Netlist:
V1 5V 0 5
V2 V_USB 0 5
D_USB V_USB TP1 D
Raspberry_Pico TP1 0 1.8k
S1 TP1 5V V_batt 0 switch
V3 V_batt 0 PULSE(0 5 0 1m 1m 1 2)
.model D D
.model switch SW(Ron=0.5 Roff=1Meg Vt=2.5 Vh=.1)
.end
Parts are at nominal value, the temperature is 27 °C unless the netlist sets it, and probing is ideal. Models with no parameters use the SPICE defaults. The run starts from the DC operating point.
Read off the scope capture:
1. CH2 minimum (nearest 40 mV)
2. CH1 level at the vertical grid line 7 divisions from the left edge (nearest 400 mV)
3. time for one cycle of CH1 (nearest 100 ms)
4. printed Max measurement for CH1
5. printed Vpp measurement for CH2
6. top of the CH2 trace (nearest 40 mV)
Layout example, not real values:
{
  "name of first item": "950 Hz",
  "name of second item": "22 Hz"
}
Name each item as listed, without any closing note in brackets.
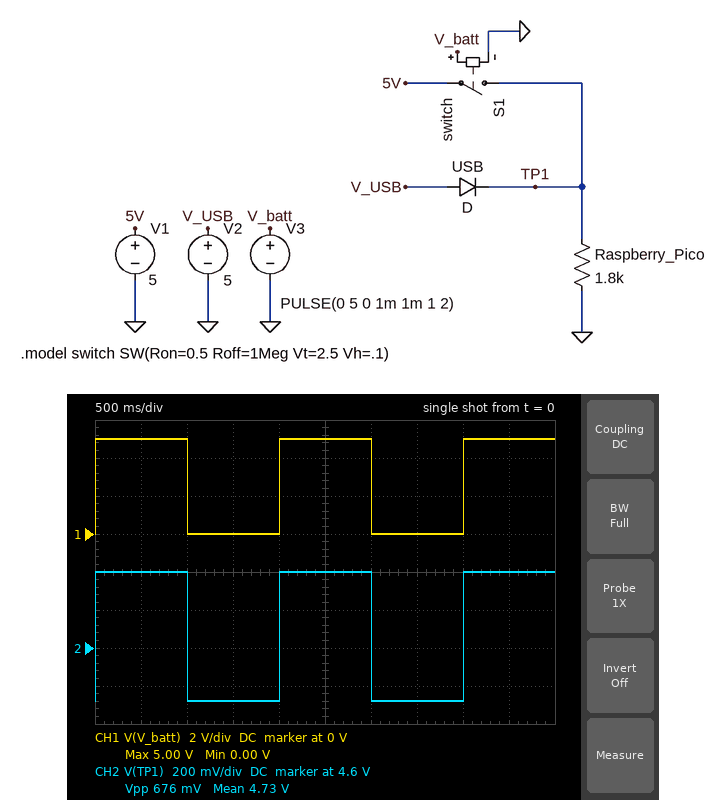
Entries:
{
  "CH2 minimum": "4.32 V",
  "CH1 level at the vertical grid line 7 divisions from the left edge": "0 V",
  "time for one cycle of CH1": "2.0 s",
  "printed Max measurement for CH1": "5.00 V",
  "printed Vpp measurement for CH2": "676 mV",
  "top of the CH2 trace": "5.00 V"
}
